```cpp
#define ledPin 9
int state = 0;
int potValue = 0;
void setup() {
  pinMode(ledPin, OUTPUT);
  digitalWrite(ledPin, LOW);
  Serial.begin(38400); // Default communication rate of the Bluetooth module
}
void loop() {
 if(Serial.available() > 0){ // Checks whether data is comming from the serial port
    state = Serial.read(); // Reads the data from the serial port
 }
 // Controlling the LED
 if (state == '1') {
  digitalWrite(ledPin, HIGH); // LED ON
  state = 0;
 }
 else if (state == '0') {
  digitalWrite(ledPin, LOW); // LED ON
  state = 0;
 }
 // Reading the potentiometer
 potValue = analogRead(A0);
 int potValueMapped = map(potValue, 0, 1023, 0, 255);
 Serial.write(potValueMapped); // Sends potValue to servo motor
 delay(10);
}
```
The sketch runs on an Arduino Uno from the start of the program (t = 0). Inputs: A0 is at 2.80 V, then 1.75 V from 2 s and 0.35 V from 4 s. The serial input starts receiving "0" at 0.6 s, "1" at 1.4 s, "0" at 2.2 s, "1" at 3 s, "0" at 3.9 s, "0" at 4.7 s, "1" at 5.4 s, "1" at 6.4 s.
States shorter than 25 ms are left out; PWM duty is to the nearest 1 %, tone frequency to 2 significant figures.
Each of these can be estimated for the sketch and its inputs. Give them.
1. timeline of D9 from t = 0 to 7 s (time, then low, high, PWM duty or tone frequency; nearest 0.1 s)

0 s low; 1.4 s high; 2.2 s low; 3 s high; 3.9 s low; 5.4 s high
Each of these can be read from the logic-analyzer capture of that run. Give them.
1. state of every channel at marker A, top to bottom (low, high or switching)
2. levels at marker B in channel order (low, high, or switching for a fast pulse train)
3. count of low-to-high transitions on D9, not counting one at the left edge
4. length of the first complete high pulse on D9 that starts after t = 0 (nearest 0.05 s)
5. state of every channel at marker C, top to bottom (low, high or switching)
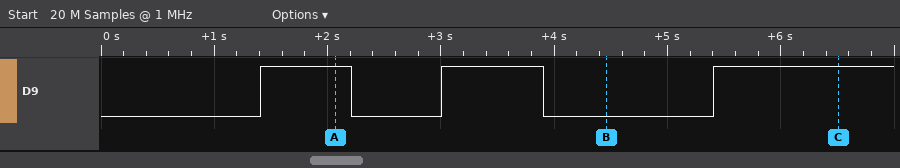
D9 high
D9 low
3
0.80 s
D9 high
